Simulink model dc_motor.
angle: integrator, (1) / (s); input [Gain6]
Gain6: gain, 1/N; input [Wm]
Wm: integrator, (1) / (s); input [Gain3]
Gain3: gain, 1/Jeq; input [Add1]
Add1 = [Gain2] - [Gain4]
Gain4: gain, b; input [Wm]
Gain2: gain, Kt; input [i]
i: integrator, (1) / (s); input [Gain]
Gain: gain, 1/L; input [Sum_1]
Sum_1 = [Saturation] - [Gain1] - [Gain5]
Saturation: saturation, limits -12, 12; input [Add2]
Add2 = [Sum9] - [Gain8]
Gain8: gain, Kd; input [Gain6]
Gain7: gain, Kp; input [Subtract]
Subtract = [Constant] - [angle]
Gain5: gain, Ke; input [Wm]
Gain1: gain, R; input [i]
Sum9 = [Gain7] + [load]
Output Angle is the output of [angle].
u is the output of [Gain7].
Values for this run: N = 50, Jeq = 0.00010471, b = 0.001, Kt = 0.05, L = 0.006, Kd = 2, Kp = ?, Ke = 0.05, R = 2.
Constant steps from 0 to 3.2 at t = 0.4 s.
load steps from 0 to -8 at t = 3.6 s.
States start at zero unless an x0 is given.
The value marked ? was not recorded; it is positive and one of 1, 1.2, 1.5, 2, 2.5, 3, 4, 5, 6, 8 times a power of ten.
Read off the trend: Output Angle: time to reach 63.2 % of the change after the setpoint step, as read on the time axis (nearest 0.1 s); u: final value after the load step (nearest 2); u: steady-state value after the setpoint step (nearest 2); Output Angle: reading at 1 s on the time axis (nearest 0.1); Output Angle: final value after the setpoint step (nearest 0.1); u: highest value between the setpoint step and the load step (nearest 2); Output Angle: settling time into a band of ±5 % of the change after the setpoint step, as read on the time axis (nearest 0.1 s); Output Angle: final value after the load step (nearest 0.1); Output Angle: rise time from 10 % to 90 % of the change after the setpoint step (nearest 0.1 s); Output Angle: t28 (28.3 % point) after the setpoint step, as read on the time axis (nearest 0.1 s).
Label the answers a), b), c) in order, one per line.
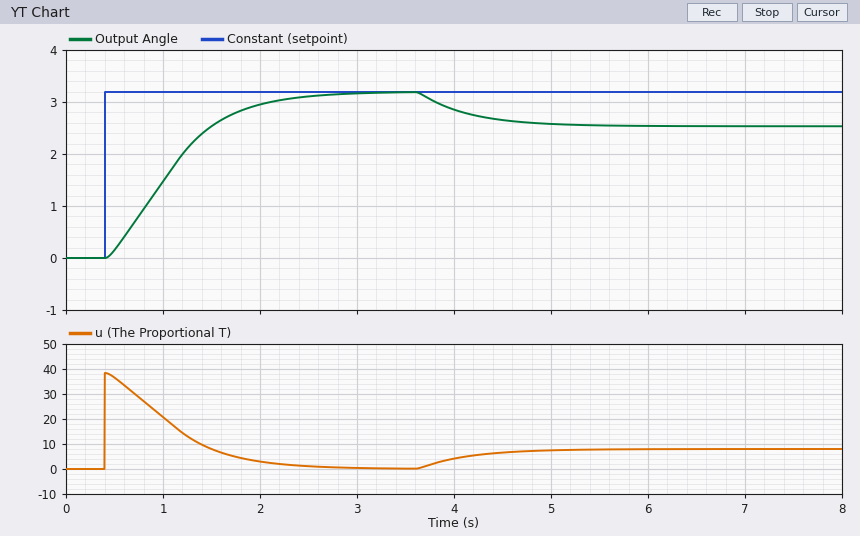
a) 1.2 s
b) 8
c) 0
d) 1.5
e) 3.2
f) 38
g) 2.2 s
h) 2.5
i) 1.3 s
j) 0.8 s
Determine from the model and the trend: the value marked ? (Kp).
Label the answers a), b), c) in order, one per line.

a) 12
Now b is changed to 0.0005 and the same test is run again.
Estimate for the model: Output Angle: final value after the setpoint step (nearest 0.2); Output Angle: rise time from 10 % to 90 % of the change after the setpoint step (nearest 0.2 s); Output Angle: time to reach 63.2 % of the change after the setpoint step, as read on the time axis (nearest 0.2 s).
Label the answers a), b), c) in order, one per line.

a) 3.2
b) 1.0 s
c) 1.0 s
